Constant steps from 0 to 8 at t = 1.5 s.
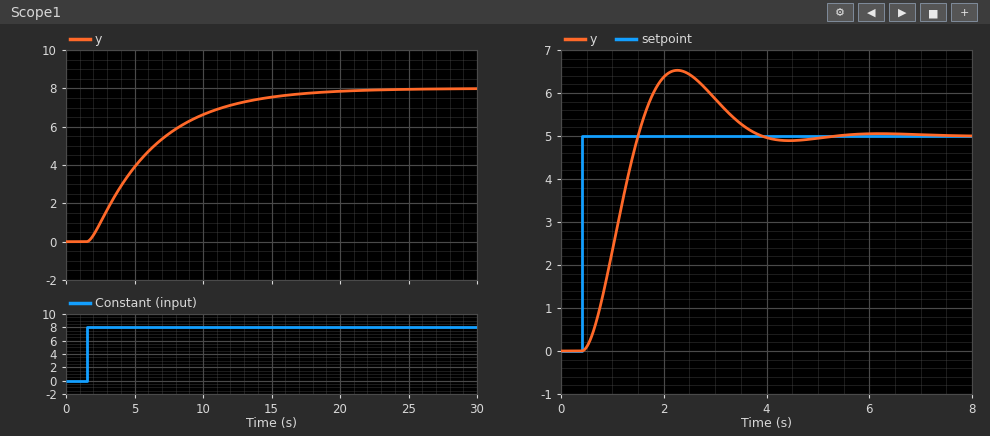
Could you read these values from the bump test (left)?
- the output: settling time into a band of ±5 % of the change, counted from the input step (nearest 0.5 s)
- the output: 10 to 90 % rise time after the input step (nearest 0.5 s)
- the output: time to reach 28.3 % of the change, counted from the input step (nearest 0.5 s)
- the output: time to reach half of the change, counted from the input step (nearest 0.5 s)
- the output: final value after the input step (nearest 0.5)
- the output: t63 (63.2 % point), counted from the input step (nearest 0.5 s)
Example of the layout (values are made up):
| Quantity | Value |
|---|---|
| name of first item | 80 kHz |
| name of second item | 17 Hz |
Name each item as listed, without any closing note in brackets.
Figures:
| Quantity | Value |
|---|---|
| the output: settling time into a band of ±5 % of the change, counted from the input step | 14.0 s |
| the output: 10 to 90 % rise time after the input step | 10.0 s |
| the output: time to reach 28.3 % of the change, counted from the input step | 2.0 s |
| the output: time to reach half of the change, counted from the input step | 3.5 s |
| the output: final value after the input step | 8.0 |
| the output: t63 (63.2 % point), counted from the input step | 5.0 s |
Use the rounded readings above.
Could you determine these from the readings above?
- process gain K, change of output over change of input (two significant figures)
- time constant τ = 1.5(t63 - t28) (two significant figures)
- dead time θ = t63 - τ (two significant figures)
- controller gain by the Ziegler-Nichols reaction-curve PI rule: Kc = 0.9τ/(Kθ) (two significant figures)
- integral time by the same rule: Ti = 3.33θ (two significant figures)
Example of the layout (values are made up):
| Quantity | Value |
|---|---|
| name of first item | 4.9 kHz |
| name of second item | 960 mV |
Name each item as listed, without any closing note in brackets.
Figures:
| Quantity | Value |
|---|---|
| process gain K, change of output over change of input | 1.0 |
| time constant τ = 1.5(t63 - t28) | 4.5 s |
| dead time θ = t63 - τ | 0.50 s |
| controller gain by the Ziegler-Nichols reaction-curve PI rule: Kc = 0.9τ/(Kθ) | 8.1 |
| integral time by the same rule: Ti = 3.33θ | 1.7 s |
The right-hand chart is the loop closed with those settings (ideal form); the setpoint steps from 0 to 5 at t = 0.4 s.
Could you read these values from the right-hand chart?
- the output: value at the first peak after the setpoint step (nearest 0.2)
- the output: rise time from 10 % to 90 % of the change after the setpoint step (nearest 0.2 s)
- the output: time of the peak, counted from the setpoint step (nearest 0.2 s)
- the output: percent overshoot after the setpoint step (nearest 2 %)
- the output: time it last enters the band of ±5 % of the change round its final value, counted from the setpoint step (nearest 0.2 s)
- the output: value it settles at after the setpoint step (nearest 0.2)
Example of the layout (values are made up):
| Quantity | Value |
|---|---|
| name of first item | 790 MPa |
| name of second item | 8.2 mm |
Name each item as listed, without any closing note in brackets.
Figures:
| Quantity | Value |
|---|---|
| the output: value at the first peak after the setpoint step | 6.6 |
| the output: rise time from 10 % to 90 % of the change after the setpoint step | 0.8 s |
| the output: time of the peak, counted from the setpoint step | 1.8 s |
| the output: percent overshoot after the setpoint step | 30 % |
| the output: time it last enters the band of ±5 % of the change round its final value, counted from the setpoint step | 3.2 s |
| the output: value it settles at after the setpoint step | 5.0 |
